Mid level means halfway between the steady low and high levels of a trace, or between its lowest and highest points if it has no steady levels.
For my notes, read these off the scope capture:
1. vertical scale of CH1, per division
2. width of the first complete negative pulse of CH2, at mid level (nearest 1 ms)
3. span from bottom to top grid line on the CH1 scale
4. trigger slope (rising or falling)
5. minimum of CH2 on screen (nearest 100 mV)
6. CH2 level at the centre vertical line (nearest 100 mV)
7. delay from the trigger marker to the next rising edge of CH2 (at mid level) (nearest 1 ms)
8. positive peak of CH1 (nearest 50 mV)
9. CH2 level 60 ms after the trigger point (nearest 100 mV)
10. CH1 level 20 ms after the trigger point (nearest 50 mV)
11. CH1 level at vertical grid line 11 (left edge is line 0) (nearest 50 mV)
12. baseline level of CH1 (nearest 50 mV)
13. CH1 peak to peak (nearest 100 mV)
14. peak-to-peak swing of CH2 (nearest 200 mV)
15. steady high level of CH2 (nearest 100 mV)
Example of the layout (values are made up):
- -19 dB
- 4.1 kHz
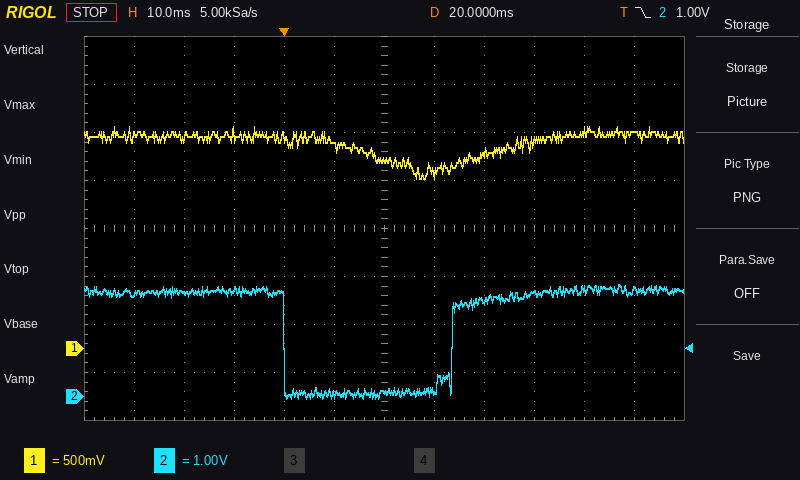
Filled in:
- 500 mV
- 34 ms
- 4 V
- falling
- 0.0 V
- 100 mV
- 34 ms
- 2.30 V
- 2.2 V
- 1.95 V
- 2.25 V
- 2.20 V
- 500 mV
- 2.4 V
- 2.2 V
